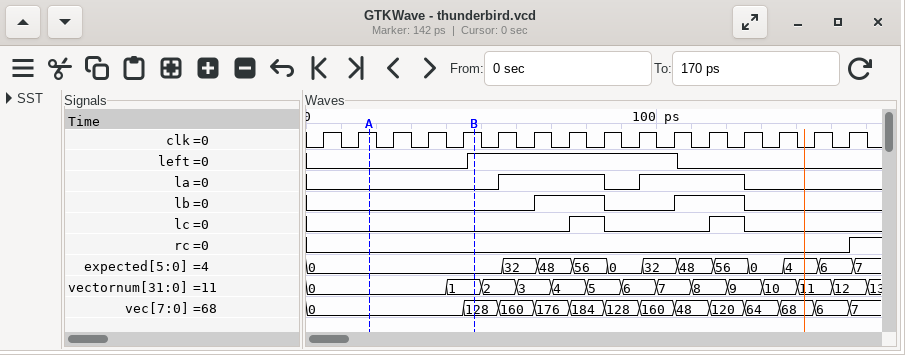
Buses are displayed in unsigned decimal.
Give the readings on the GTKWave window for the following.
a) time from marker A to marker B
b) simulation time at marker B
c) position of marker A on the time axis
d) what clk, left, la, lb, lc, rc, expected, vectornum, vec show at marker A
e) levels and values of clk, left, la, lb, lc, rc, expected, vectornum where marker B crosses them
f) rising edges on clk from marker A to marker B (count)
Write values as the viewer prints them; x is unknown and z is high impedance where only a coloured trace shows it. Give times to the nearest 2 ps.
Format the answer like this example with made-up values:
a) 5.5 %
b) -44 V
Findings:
a) 30 ps
b) 48 ps
c) 18 ps
d) clk=1, left=0, la=0, lb=0, lc=0, rc=0, expected=0, vectornum=0, vec=0
e) clk=1, left=1, la=0, lb=0, lc=0, rc=0, expected=0, vectornum=1
f) 3
